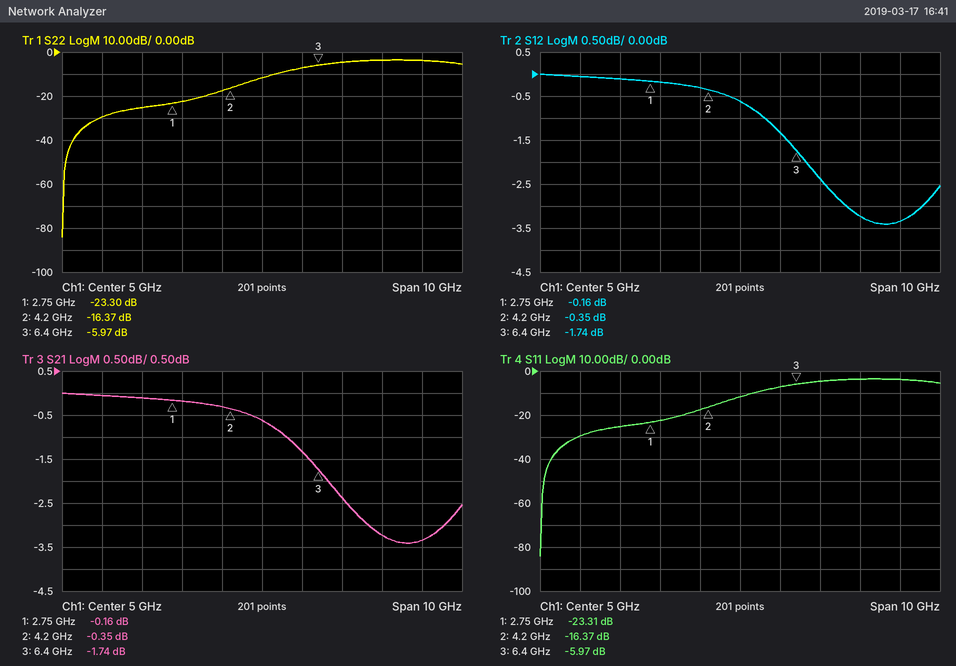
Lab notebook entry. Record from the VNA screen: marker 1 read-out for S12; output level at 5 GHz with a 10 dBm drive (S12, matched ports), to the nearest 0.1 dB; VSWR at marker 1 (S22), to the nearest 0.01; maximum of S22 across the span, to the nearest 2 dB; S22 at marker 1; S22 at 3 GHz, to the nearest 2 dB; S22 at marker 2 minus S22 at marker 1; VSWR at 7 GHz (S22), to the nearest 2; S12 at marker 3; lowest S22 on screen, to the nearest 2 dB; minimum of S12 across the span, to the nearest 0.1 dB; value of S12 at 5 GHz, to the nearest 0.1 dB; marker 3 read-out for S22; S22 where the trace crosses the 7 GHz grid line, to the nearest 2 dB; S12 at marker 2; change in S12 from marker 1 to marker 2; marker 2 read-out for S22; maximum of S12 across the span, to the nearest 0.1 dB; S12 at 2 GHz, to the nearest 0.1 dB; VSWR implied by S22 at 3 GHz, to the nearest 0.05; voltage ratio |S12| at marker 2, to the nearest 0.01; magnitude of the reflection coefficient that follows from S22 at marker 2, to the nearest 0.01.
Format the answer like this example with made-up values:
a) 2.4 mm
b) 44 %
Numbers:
a) -0.16 dB
b) 9.4 dBm
c) 1.15
d) -4 dB
e) -23.30 dB
f) -22 dB
g) 6.93 dB
h) 4
i) -1.74 dB
j) -84 dB
k) -3.4 dB
l) -0.6 dB
m) -5.97 dB
n) -4 dB
o) -0.35 dB
p) -0.19 dB
q) -16.37 dB
r) 0.0 dB
s) -0.1 dB
t) 1.15
u) 0.96
v) 0.15
